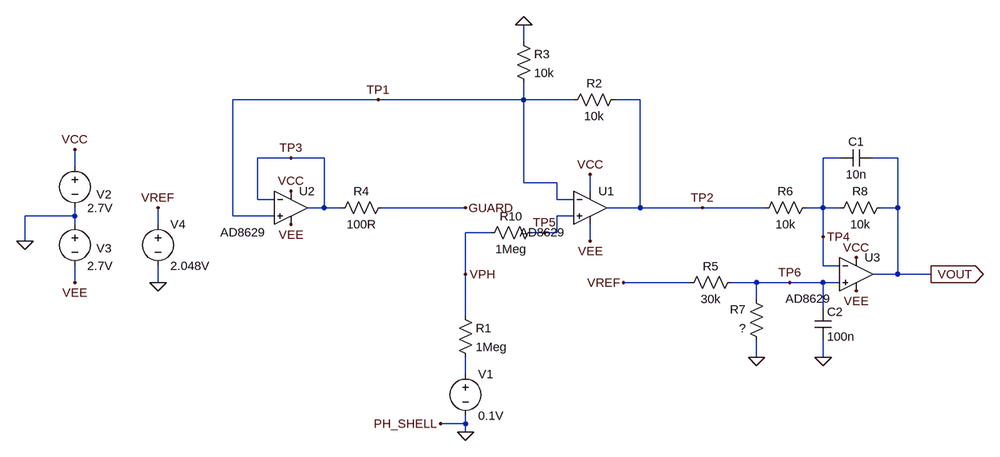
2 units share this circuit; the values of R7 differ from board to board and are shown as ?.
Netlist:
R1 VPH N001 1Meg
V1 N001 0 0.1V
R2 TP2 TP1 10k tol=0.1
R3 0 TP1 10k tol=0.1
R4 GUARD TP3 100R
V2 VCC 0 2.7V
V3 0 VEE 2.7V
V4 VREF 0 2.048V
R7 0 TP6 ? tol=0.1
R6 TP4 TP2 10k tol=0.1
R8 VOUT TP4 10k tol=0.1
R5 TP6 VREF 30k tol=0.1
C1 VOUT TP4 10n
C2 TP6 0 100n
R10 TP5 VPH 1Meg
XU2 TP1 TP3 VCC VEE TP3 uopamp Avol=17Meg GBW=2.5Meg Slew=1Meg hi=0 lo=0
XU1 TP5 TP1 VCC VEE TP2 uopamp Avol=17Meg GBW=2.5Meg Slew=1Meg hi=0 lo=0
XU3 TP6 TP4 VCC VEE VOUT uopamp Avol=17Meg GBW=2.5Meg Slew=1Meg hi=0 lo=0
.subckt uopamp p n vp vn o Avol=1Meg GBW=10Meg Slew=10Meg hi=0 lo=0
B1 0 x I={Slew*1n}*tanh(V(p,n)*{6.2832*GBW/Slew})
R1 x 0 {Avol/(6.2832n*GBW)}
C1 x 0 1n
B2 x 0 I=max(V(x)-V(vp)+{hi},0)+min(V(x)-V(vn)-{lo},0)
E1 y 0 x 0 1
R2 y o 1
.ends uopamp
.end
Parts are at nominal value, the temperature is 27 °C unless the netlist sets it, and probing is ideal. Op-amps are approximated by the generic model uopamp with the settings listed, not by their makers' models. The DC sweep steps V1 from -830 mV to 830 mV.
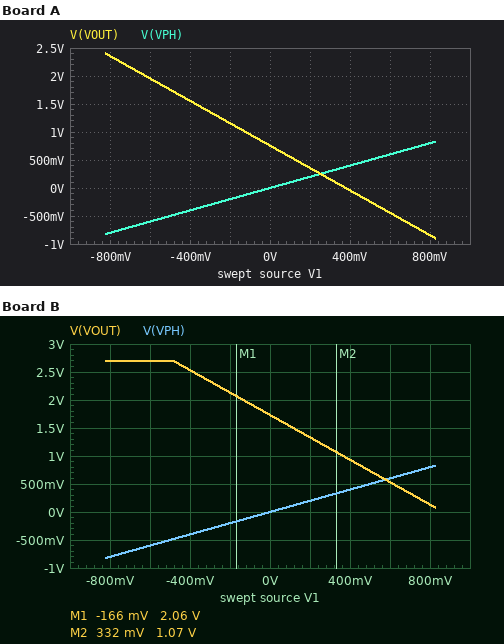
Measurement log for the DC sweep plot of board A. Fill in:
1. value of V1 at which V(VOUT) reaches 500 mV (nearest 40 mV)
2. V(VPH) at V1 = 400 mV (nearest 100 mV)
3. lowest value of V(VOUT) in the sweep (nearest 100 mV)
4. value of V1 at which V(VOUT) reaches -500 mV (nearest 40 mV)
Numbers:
120 mV
400 mV
-900 mV
640 mV
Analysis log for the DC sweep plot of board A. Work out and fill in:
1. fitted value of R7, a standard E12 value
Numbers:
6.8 kΩ
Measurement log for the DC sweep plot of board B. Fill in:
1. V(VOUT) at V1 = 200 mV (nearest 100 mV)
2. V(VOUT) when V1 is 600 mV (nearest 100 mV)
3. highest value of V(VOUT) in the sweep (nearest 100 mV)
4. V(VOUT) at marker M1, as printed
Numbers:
1.3 V
500 mV
2.7 V
2.06 V
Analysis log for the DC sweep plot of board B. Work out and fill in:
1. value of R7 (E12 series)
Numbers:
22 kΩ
